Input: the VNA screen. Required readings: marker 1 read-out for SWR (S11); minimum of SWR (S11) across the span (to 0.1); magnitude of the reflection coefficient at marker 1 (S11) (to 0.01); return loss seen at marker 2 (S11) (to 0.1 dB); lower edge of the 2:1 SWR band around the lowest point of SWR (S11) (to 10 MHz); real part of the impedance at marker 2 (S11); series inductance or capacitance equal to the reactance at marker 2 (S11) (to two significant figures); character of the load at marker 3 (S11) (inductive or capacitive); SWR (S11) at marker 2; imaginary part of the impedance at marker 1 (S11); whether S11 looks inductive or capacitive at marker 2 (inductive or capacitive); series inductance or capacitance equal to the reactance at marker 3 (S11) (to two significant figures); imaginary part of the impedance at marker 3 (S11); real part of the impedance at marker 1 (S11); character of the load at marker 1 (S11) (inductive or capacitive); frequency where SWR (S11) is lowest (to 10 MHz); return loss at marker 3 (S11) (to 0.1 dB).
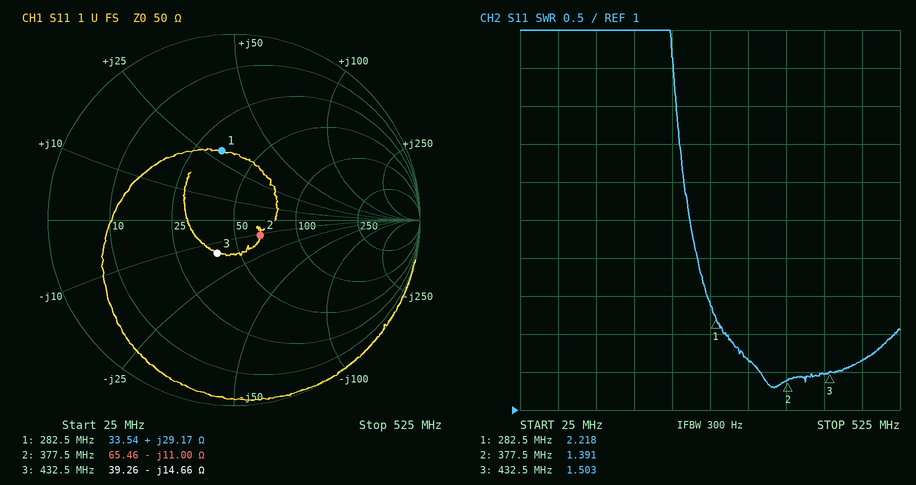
2.218
1.3
0.38
15.7 dB
300 MHz
65.46 Ω
38 pF
capacitive
1.391
+29.17 Ω
capacitive
25 pF
-14.66 Ω
33.54 Ω
inductive
360 MHz
13.9 dB
